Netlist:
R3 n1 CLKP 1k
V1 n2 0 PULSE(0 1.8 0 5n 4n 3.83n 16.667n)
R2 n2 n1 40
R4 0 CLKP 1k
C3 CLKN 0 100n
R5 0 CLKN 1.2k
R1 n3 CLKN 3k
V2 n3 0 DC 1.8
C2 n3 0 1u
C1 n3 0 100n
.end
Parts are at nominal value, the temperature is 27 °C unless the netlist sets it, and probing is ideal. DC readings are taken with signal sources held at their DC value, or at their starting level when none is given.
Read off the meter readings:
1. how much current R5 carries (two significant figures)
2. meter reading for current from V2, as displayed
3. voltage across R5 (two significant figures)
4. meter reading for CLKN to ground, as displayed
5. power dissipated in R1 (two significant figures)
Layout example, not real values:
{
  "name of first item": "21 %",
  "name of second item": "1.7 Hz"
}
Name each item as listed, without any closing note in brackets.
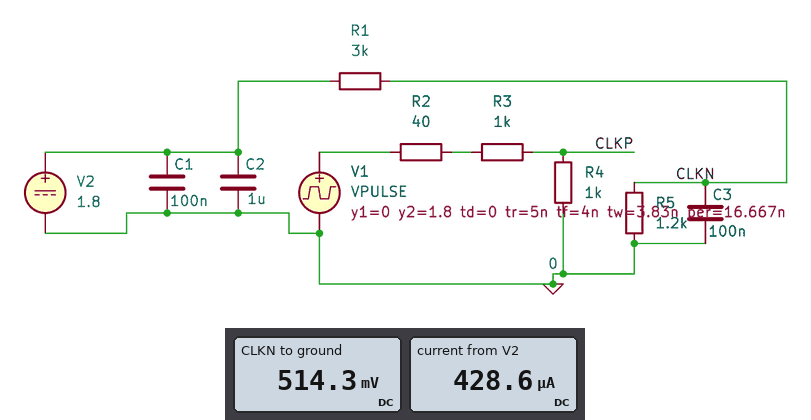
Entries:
{
  "how much current R5 carries": "430 µA",
  "meter reading for current from V2, as displayed": "428.6 µA",
  "voltage across R5": "510 mV",
  "meter reading for CLKN to ground, as displayed": "514.3 mV",
  "power dissipated in R1": "550 µW"
}
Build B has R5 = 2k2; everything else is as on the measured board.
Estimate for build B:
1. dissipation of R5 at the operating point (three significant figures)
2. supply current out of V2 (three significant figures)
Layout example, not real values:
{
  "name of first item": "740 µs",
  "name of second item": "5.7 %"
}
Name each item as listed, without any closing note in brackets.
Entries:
{
  "dissipation of R5 at the operating point": "264 µW",
  "supply current out of V2": "346 µA"
}
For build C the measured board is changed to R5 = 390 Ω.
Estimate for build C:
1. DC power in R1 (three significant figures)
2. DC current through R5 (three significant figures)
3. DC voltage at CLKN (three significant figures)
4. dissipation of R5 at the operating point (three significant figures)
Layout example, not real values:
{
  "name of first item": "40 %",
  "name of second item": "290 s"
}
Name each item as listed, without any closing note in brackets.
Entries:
{
  "DC power in R1": "846 µW",
  "DC current through R5": "531 µA",
  "DC voltage at CLKN": "207 mV",
  "dissipation of R5 at the operating point": "110 µW"
}
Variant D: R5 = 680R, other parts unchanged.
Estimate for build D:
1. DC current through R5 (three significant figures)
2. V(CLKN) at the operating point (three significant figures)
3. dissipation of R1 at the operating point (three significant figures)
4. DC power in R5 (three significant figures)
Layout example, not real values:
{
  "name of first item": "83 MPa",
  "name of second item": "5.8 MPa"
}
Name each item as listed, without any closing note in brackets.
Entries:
{
  "DC current through R5": "489 µA",
  "V(CLKN) at the operating point": "333 mV",
  "dissipation of R1 at the operating point": "718 µW",
  "DC power in R5": "163 µW"
}
